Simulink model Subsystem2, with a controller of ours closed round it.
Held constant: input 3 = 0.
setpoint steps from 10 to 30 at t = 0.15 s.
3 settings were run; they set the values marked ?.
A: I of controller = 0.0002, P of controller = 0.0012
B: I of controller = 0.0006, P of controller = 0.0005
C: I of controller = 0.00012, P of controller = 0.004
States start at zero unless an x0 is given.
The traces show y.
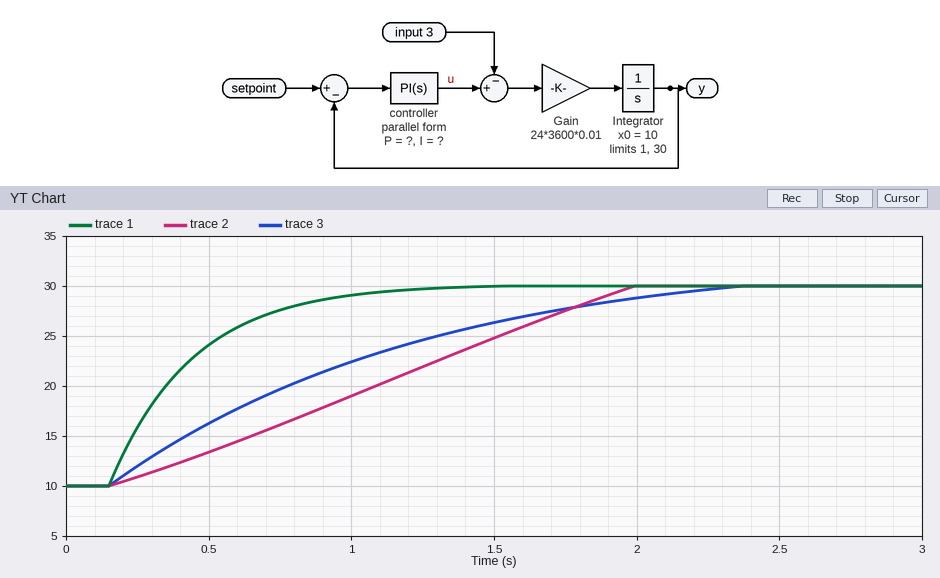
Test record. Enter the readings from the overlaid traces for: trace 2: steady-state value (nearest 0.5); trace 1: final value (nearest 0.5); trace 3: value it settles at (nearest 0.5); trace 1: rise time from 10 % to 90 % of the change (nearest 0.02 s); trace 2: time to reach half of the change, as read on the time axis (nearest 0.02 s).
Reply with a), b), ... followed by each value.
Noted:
a) 30.0
b) 30.0
c) 30.0
d) 0.62 s
e) 1.08 s
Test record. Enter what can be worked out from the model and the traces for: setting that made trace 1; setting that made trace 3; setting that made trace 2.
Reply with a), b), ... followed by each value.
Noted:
a) C
b) A
c) B
